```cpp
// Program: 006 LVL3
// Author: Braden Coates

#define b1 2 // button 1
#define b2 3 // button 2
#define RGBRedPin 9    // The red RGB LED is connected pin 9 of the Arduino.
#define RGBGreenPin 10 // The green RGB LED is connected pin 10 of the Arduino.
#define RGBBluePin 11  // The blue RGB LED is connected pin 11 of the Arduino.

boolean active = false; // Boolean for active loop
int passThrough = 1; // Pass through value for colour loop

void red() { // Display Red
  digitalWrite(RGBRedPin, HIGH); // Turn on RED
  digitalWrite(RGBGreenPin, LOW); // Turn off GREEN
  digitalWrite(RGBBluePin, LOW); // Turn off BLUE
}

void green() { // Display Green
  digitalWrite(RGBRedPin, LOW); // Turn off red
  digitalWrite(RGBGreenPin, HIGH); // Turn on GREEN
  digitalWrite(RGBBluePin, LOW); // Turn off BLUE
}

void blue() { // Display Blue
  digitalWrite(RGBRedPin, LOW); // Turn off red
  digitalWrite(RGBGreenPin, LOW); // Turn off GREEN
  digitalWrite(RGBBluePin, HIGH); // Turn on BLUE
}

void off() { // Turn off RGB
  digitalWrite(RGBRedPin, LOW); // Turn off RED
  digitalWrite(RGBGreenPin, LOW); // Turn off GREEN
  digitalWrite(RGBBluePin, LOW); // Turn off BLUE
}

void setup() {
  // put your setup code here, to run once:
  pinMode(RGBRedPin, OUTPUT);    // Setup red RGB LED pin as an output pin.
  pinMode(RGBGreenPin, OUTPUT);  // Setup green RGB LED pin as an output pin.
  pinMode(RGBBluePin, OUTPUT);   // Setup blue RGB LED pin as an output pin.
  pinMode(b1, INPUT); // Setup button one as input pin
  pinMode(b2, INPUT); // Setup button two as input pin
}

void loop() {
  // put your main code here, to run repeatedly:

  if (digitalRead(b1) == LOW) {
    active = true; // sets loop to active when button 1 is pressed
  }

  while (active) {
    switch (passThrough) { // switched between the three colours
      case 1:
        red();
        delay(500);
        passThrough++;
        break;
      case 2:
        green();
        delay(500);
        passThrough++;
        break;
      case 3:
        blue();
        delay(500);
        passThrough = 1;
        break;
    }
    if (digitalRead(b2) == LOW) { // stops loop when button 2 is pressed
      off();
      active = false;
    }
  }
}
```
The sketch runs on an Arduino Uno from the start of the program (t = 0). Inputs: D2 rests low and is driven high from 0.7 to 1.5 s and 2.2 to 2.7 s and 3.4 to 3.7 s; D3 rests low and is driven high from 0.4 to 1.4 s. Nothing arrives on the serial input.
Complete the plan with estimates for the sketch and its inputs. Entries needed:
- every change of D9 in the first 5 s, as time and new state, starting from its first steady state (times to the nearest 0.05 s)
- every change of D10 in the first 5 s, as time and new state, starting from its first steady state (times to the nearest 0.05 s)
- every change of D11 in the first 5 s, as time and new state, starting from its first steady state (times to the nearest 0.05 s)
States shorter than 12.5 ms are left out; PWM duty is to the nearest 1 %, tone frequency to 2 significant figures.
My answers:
0 s high; 0.5 s low; 1.5 s high; 2 s low; 3.2 s high; 3.7 s low; 4.7 s high
0 s low; 0.5 s high; 1 s low; 2 s high; 2.5 s low; 3.7 s high; 4.2 s low
0 s low; 1 s high; 1.5 s low; 2.7 s high; 3.2 s low; 4.2 s high; 4.7 s low
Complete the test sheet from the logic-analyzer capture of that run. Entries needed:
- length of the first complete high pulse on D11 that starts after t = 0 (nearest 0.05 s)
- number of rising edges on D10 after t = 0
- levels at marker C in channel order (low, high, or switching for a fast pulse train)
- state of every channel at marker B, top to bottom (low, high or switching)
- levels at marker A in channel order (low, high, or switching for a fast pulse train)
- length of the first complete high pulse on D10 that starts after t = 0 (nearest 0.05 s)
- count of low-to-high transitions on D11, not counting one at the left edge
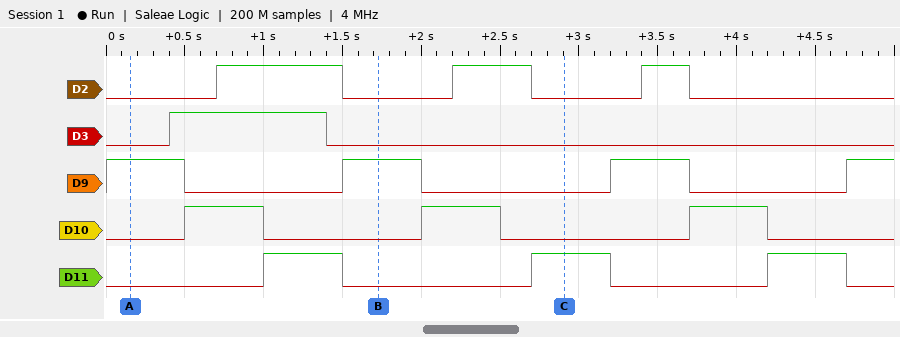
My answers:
0.50 s
3
D2 low, D3 low, D9 low, D10 low, D11 high
D2 low, D3 low, D9 high, D10 low, D11 low
D2 low, D3 low, D9 high, D10 low, D11 low
0.50 s
3
